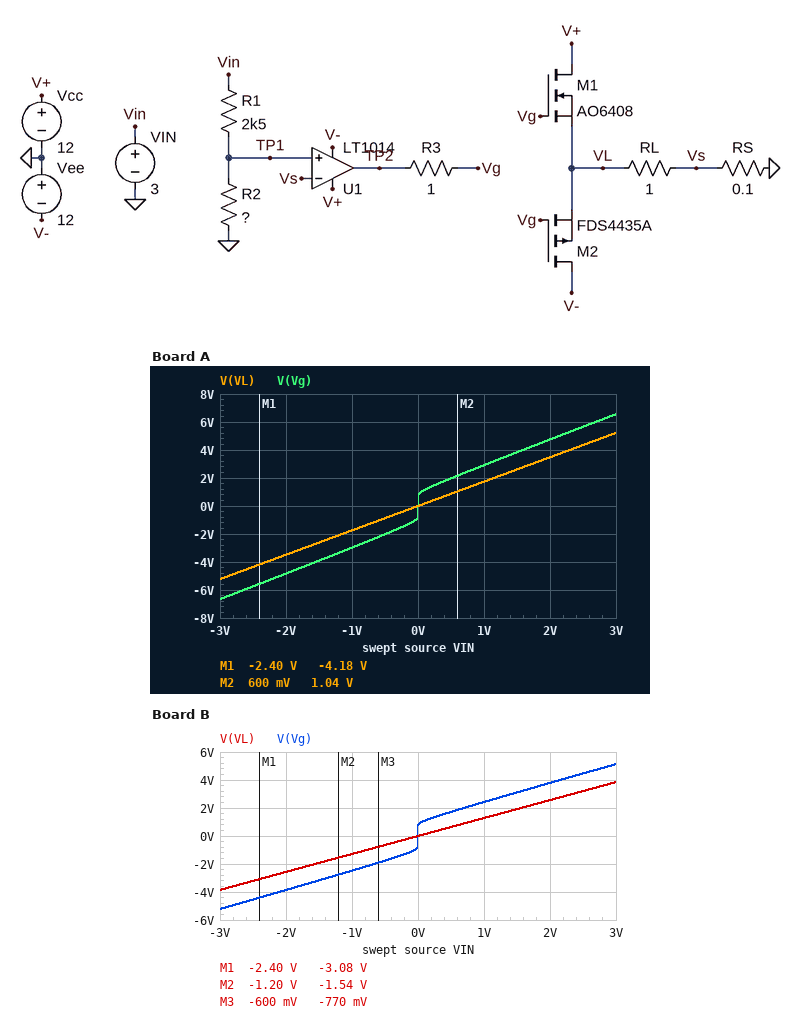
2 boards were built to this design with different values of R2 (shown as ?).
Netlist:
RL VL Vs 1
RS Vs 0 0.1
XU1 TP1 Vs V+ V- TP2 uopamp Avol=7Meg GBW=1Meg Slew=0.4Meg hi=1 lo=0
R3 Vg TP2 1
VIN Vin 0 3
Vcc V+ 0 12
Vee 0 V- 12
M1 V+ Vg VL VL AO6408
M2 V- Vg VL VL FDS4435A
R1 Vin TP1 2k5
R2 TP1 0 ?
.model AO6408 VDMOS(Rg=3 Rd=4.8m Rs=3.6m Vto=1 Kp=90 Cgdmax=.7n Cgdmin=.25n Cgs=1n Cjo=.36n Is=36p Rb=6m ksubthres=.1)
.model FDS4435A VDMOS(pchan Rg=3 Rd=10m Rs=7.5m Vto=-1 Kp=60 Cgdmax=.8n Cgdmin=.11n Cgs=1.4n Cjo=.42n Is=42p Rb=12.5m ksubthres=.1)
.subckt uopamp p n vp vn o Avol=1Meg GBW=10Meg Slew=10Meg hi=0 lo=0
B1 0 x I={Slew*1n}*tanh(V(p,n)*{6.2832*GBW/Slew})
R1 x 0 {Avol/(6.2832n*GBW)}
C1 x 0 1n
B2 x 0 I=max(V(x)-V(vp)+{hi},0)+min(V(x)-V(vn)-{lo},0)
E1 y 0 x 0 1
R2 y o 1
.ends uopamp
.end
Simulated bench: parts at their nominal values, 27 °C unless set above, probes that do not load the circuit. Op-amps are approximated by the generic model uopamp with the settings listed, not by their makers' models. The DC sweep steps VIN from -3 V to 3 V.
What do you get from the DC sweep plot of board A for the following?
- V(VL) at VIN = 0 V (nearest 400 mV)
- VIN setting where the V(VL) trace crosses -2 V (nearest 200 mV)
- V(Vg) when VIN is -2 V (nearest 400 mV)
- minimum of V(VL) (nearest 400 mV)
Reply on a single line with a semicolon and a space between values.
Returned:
0 V; -1.2 V; -4.8 V; -5.2 V
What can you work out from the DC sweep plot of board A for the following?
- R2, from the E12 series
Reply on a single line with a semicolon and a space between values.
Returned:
470 Ω
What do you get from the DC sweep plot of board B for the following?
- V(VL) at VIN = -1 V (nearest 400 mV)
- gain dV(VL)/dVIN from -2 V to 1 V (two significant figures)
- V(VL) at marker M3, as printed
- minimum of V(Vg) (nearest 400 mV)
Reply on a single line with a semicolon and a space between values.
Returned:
-1.2 V; 1.3 V/V; -770 mV; -5.2 V
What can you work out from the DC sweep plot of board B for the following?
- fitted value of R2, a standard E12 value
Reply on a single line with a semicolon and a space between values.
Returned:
330 Ω
